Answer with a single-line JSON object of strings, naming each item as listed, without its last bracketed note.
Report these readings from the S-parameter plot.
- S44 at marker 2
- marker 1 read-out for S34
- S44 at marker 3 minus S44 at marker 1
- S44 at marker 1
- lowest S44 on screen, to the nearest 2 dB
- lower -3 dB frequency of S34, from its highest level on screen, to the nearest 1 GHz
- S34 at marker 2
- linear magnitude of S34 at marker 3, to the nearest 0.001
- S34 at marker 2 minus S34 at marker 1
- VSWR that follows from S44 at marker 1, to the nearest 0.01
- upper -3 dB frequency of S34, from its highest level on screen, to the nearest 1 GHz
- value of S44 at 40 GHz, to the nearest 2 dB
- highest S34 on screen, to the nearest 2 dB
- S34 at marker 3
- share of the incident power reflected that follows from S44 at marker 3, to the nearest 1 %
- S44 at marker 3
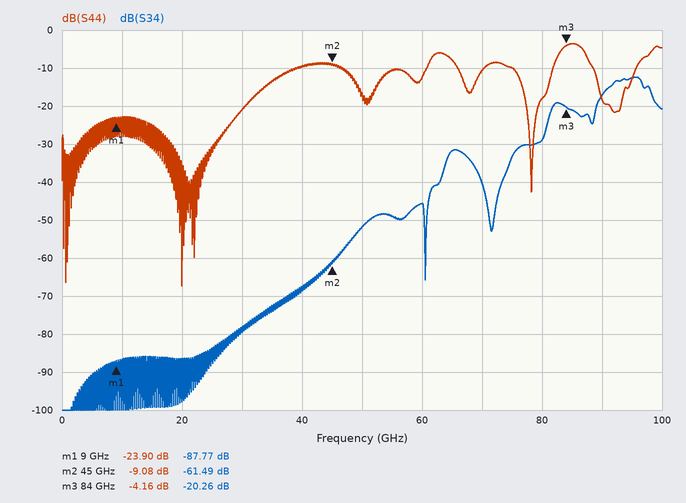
{"S44 at marker 2": "-9.08 dB", "marker 1 read-out for S34": "-87.77 dB", "S44 at marker 3 minus S44 at marker 1": "19.74 dB", "S44 at marker 1": "-23.90 dB", "lowest S44 on screen, to the nearest 2 dB": "-68 dB", "lower -3 dB frequency of S34, from its highest level on screen, to the nearest 1 GHz": "91 GHz", "S34 at marker 2": "-61.49 dB", "linear magnitude of S34 at marker 3, to the nearest 0.001": "0.097", "S34 at marker 2 minus S34 at marker 1": "26.28 dB", "VSWR that follows from S44 at marker 1, to the nearest 0.01": "1.14", "upper -3 dB frequency of S34, from its highest level on screen, to the nearest 1 GHz": "98 GHz", "value of S44 at 40 GHz, to the nearest 2 dB": "-10 dB", "highest S34 on screen, to the nearest 2 dB": "-12 dB", "S34 at marker 3": "-20.26 dB", "share of the incident power reflected that follows from S44 at marker 3, to the nearest 1 %": "38 %", "S44 at marker 3": "-4.16 dB"}
